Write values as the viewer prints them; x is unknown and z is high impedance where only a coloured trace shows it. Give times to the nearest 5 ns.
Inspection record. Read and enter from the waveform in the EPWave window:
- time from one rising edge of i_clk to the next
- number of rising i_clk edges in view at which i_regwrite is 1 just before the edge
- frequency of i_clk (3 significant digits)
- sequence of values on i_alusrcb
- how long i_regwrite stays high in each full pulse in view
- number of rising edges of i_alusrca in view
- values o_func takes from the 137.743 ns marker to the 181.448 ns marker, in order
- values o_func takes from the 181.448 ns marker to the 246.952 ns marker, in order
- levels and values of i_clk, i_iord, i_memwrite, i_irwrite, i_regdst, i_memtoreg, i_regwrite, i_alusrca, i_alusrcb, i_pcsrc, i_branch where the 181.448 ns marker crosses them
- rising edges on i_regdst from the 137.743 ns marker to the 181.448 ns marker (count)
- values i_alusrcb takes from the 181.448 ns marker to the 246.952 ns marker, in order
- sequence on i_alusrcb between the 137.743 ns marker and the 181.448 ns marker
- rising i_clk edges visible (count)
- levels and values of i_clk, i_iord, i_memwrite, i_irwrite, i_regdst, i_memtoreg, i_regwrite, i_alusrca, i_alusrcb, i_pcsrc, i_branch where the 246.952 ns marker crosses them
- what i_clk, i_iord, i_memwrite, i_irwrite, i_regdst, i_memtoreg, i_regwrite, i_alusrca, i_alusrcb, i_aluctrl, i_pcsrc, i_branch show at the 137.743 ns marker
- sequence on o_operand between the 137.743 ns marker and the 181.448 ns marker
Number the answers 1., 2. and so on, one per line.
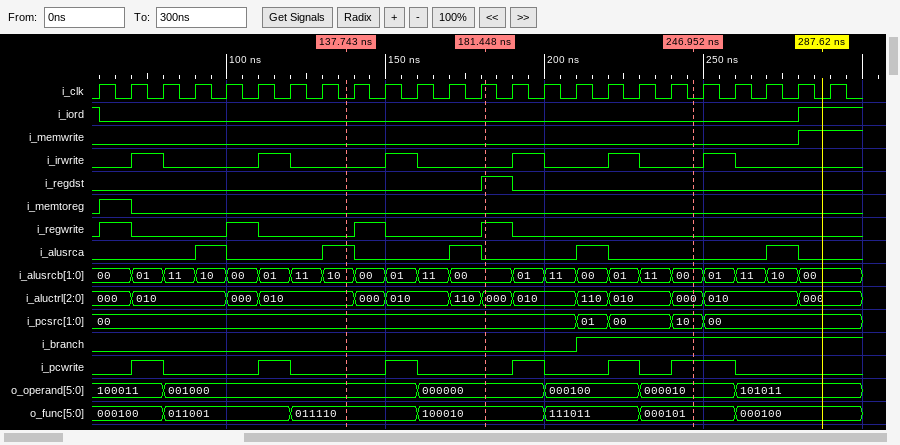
1. 10 ns
2. 4
3. 100 MHz
4. 00, 01, 11, 10, 00, 01, 11, 10, 00, 01, 11, 00, 01, 11, 00, 01, 11, 00, 01, 11, 10, 00
5. 10 ns, 10 ns, 10 ns, 10 ns
6. 5
7. 011110, 100010
8. 100010, 111011, 000101
9. i_clk=1, i_iord=0, i_memwrite=0, i_irwrite=0, i_regdst=1, i_memtoreg=0, i_regwrite=1, i_alusrca=0, i_alusrcb=00, i_pcsrc=00, i_branch=0
10. 1
11. 00, 01, 11, 00, 01, 11, 00
12. 10, 00, 01, 11, 00
13. 24
14. i_clk=0, i_iord=0, i_memwrite=0, i_irwrite=0, i_regdst=0, i_memtoreg=0, i_regwrite=0, i_alusrca=0, i_alusrcb=00, i_pcsrc=10, i_branch=1
15. i_clk=0, i_iord=0, i_memwrite=0, i_irwrite=0, i_regdst=0, i_memtoreg=0, i_regwrite=0, i_alusrca=1, i_alusrcb=10, i_aluctrl=010, i_pcsrc=00, i_branch=0
16. 001000, 000000
